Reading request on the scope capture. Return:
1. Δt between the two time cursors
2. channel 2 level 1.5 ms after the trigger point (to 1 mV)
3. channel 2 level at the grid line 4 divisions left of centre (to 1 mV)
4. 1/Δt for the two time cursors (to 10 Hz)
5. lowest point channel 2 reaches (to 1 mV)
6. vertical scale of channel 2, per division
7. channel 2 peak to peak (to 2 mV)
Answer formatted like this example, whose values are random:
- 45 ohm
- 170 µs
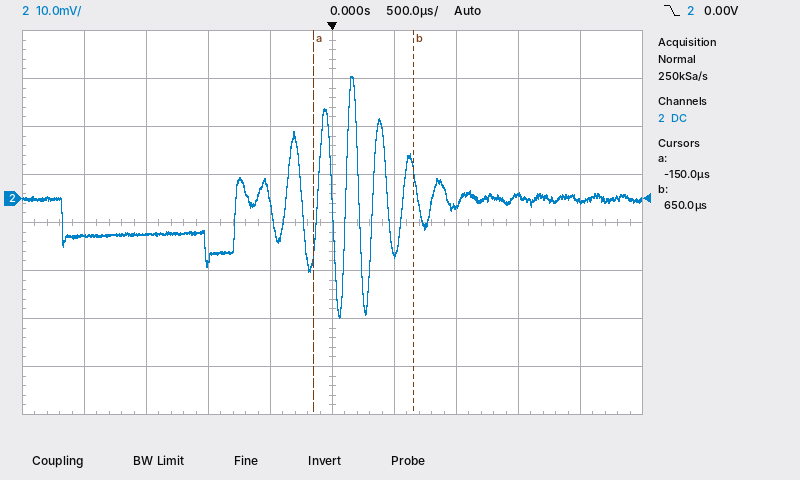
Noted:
- 800 µs
- 1 mV
- -8 mV
- 1.25 kHz
- -25 mV
- 10 mV
- 50 mV
